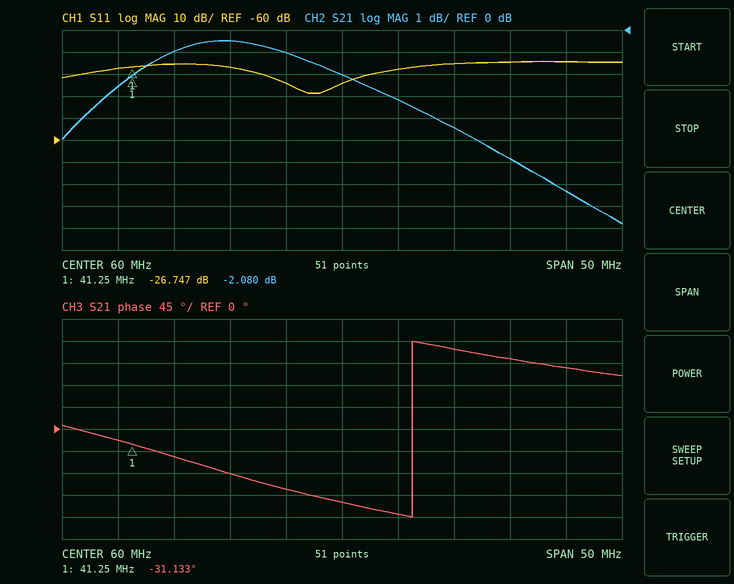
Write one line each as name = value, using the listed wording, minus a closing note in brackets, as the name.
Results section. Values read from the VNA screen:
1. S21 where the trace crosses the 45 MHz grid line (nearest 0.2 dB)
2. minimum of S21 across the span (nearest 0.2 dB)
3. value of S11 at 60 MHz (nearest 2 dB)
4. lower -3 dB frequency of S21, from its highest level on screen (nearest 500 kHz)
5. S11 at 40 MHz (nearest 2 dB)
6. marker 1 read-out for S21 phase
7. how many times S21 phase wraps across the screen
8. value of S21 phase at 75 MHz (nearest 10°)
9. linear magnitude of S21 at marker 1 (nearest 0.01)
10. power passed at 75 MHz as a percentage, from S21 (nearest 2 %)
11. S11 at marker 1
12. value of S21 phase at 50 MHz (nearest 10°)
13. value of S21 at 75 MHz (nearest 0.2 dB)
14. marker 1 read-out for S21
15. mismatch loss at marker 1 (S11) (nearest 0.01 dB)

S21 where the trace crosses the 45 MHz grid line = -1.0 dB
minimum of S21 across the span = -8.8 dB
value of S11 at 60 MHz = -34 dB
lower -3 dB frequency of S21, from its highest level on screen = 38.0 MHz
S11 at 40 MHz = -28 dB
marker 1 read-out for S21 phase = -31.133°
how many times S21 phase wraps across the screen = 1
value of S21 phase at 75 MHz = 140°
linear magnitude of S21 at marker 1 = 0.79
power passed at 75 MHz as a percentage, from S21 = 26 %
S11 at marker 1 = -26.747 dB
value of S21 phase at 50 MHz = -90°
value of S21 at 75 MHz = -5.8 dB
marker 1 read-out for S21 = -2.080 dB
mismatch loss at marker 1 (S11) = 0.01 dB
